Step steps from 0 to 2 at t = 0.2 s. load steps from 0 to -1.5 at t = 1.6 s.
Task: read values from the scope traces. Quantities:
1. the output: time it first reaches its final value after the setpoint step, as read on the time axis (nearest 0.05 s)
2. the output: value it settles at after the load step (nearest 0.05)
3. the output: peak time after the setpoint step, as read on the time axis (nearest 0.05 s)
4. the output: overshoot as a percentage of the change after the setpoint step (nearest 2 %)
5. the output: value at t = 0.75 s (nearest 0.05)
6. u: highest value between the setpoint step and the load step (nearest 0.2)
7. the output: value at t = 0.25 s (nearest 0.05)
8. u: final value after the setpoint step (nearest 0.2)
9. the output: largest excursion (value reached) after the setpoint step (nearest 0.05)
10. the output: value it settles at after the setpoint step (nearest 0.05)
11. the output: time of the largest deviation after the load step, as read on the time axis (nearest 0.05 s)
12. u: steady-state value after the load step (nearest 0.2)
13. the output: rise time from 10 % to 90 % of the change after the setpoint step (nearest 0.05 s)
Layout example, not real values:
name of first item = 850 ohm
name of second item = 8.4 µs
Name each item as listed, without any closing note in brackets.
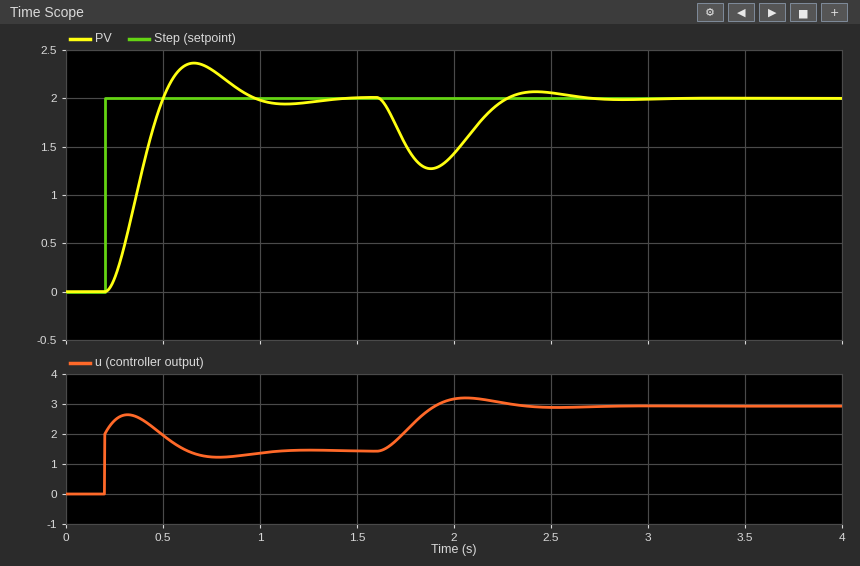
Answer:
the output: time it first reaches its final value after the setpoint step, as read on the time axis = 0.50 s
the output: value it settles at after the load step = 2.00
the output: peak time after the setpoint step, as read on the time axis = 0.65 s
the output: overshoot as a percentage of the change after the setpoint step = 18 %
the output: value at t = 0.75 s = 2.30
u: highest value between the setpoint step and the load step = 2.6
the output: value at t = 0.25 s = 0.15
u: final value after the setpoint step = 1.4
the output: largest excursion (value reached) after the setpoint step = 2.35
the output: value it settles at after the setpoint step = 2.00
the output: time of the largest deviation after the load step, as read on the time axis = 1.90 s
u: steady-state value after the load step = 3.0
the output: rise time from 10 % to 90 % of the change after the setpoint step = 0.20 s
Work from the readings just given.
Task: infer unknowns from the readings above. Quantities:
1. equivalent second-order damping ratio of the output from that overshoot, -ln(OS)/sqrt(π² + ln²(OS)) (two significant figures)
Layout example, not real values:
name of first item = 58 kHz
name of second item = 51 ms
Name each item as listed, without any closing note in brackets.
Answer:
equivalent second-order damping ratio of the output from that overshoot, -ln(OS)/sqrt(π² + ln²(OS)) = 0.48
